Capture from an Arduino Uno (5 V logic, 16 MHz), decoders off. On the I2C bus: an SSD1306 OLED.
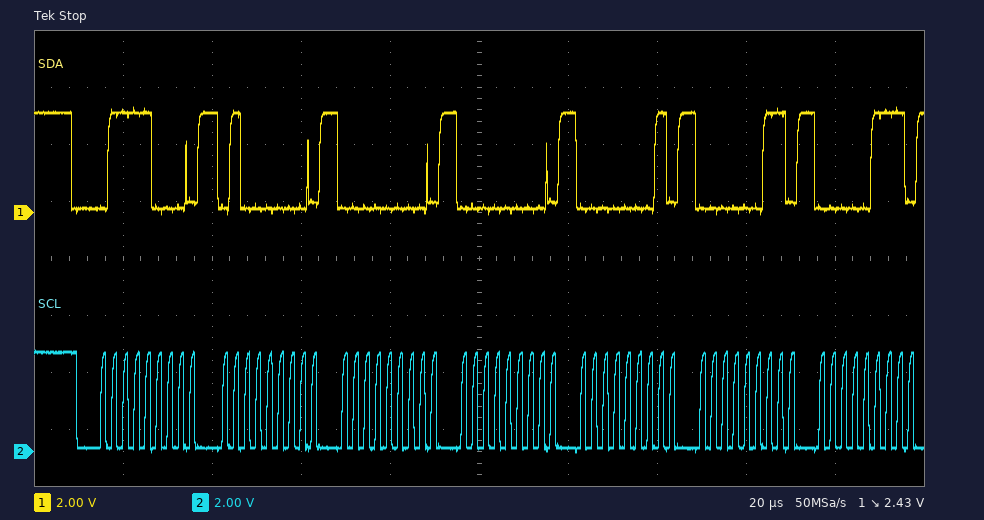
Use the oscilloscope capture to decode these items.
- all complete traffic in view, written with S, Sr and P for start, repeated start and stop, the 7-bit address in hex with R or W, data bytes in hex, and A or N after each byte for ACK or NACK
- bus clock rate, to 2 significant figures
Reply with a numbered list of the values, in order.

1. S 3CW A 40 A 00 A 00 A 01 A 03 A 07 A
2. 400 kHz
